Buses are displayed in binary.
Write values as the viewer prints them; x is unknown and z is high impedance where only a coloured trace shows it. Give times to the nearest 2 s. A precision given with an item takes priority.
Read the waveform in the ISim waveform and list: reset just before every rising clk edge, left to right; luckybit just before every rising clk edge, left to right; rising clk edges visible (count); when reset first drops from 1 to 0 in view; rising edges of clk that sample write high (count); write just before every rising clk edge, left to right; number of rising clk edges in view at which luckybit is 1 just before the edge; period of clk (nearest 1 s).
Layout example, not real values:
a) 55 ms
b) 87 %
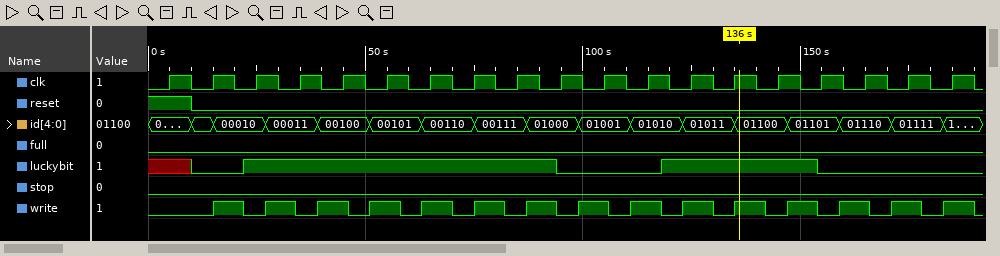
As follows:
a) 1 0 0 0 0 0 0 0 0 0 0 0 0 0 0 0 0 0 0
b) x 0 1 1 1 1 1 1 1 0 0 0 1 1 1 0 0 0 0
c) 19
d) 10 s
e) 9
f) 0 0 0 0 1 1 1 0 0 0 1 1 1 0 0 0 1 1 1
g) 10
h) 10 s
